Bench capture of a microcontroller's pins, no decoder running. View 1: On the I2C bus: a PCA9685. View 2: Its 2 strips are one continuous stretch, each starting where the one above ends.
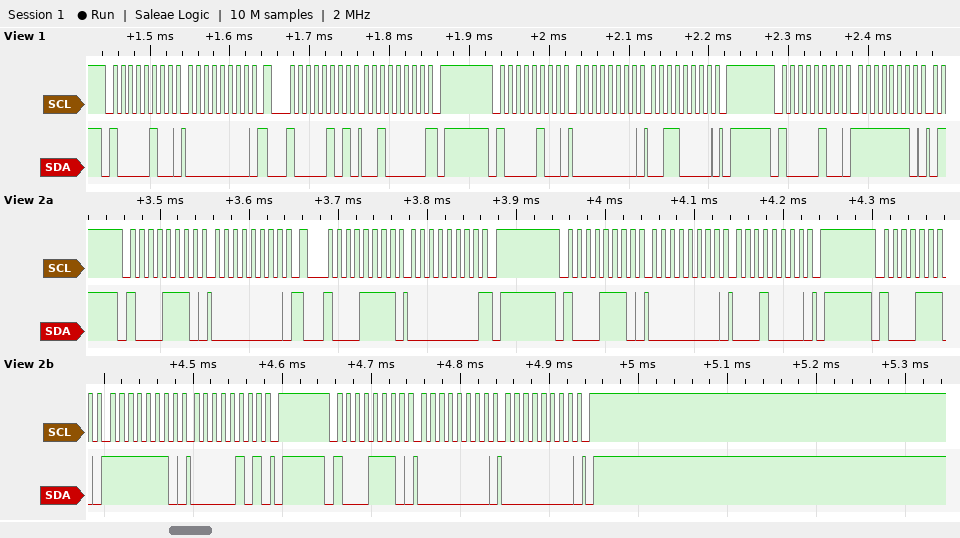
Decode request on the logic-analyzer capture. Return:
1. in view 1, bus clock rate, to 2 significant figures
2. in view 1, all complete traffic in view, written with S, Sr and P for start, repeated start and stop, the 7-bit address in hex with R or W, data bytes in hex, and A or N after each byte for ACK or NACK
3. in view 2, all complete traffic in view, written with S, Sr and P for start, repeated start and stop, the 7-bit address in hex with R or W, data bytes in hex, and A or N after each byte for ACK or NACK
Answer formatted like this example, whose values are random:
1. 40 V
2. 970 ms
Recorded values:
1. 100 kHz
2. S 42W A 00 A Sr 42R A 20 N P S 42W A 00 A 30 A P S 42W A FE A
3. S 47W A 00 A Sr 47R A 00 N P S 47W A 00 A 10 A P S 47W A FE A 05 A P S 47W A 00 A 00 A P
